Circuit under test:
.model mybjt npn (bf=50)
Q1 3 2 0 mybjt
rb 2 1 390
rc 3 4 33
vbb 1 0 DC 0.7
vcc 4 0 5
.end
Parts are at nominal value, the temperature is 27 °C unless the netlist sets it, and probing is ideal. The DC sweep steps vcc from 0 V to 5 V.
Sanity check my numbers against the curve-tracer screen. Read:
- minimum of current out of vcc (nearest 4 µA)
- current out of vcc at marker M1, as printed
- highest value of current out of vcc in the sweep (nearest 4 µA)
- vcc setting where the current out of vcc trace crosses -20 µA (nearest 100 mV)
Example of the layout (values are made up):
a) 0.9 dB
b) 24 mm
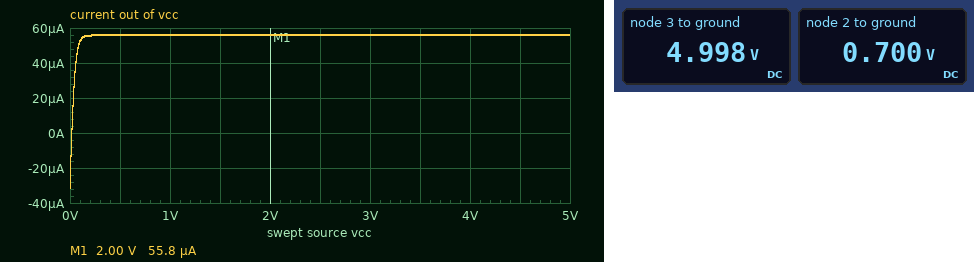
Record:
a) -32 µA
b) 55.8 µA
c) 56 µA
d) 0 V
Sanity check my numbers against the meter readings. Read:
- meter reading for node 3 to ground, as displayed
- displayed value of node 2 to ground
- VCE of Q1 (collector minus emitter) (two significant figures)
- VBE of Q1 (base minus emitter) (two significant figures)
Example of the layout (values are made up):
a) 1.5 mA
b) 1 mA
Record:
a) 4.998 V
b) 0.700 V
c) 5.0 V
d) 700 mV
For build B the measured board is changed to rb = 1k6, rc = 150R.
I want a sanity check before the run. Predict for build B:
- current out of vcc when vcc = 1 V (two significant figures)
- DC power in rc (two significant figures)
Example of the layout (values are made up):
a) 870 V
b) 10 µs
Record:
a) 53 µA
b) 420 nW
